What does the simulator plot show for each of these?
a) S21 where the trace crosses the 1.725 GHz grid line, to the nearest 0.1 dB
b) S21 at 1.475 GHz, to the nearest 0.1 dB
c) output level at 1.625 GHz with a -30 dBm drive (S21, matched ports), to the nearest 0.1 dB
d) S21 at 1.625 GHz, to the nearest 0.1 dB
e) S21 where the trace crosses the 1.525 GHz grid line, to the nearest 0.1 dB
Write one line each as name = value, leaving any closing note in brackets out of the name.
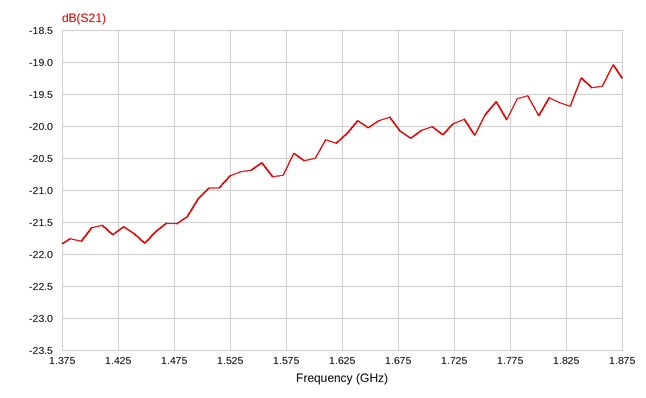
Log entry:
S21 where the trace crosses the 1.725 GHz grid line, to the nearest 0.1 dB = -20.0 dB
S21 at 1.475 GHz, to the nearest 0.1 dB = -21.5 dB
output level at 1.625 GHz with a -30 dBm drive (S21, matched ports), to the nearest 0.1 dB = -50.2 dBm
S21 at 1.625 GHz, to the nearest 0.1 dB = -20.2 dB
S21 where the trace crosses the 1.525 GHz grid line, to the nearest 0.1 dB = -20.8 dB
